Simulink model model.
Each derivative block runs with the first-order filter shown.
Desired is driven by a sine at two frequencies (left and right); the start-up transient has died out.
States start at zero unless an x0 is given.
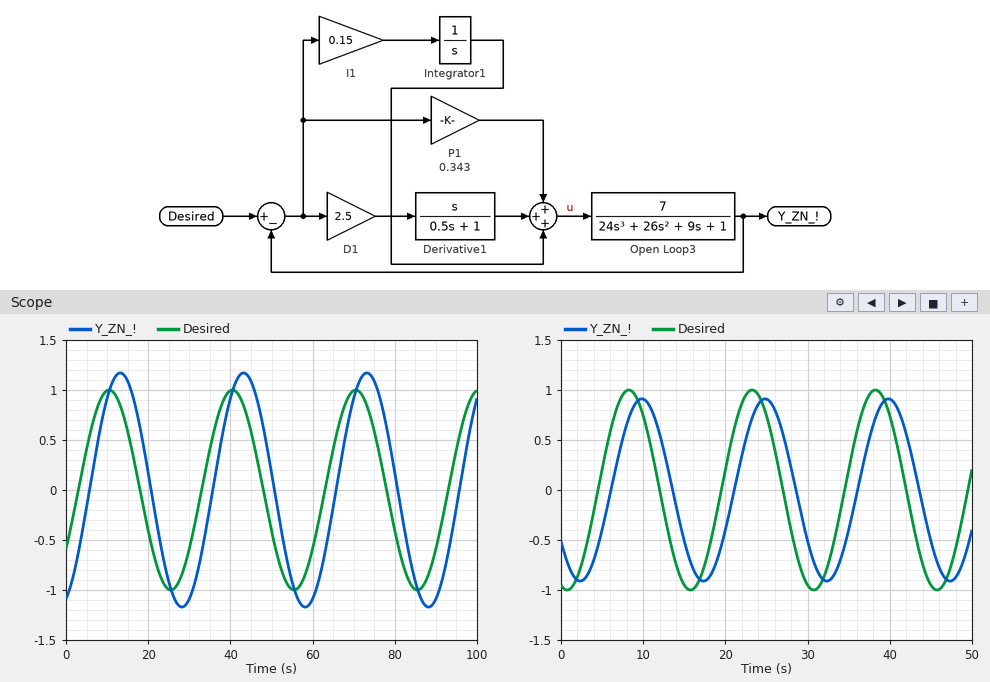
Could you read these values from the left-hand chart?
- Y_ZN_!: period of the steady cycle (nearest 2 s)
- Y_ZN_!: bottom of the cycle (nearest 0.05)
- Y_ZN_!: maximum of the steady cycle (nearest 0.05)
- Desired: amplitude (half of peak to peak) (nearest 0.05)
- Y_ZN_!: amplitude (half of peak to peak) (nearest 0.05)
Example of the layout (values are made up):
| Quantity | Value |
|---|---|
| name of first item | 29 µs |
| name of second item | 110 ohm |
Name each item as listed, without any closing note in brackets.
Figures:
| Quantity | Value |
|---|---|
| Y_ZN_!: period of the steady cycle | 30 s |
| Y_ZN_!: bottom of the cycle | -1.15 |
| Y_ZN_!: maximum of the steady cycle | 1.15 |
| Desired: amplitude (half of peak to peak) | 1.00 |
| Y_ZN_!: amplitude (half of peak to peak) | 1.15 |
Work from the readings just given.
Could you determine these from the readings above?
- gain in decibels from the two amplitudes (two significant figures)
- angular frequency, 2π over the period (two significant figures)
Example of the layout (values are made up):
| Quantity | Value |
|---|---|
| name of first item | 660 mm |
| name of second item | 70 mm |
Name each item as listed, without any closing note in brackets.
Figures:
| Quantity | Value |
|---|---|
| gain in decibels from the two amplitudes | 1.2 dB |
| angular frequency, 2π over the period | 0.21 rad/s |
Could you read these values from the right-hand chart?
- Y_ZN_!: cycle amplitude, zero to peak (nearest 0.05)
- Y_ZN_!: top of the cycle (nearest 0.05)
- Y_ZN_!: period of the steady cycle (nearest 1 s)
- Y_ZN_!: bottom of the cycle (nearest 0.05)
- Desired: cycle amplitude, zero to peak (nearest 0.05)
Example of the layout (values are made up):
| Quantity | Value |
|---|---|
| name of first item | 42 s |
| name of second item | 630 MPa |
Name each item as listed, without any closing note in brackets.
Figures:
| Quantity | Value |
|---|---|
| Y_ZN_!: cycle amplitude, zero to peak | 0.90 |
| Y_ZN_!: top of the cycle | 0.90 |
| Y_ZN_!: period of the steady cycle | 15 s |
| Y_ZN_!: bottom of the cycle | -0.90 |
| Desired: cycle amplitude, zero to peak | 1.00 |
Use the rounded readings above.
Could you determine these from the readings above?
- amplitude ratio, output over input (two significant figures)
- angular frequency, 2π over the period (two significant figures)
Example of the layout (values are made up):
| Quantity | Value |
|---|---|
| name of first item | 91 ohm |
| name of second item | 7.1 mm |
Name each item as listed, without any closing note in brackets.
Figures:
| Quantity | Value |
|---|---|
| amplitude ratio, output over input | 0.90 |
| angular frequency, 2π over the period | 0.42 rad/s |
